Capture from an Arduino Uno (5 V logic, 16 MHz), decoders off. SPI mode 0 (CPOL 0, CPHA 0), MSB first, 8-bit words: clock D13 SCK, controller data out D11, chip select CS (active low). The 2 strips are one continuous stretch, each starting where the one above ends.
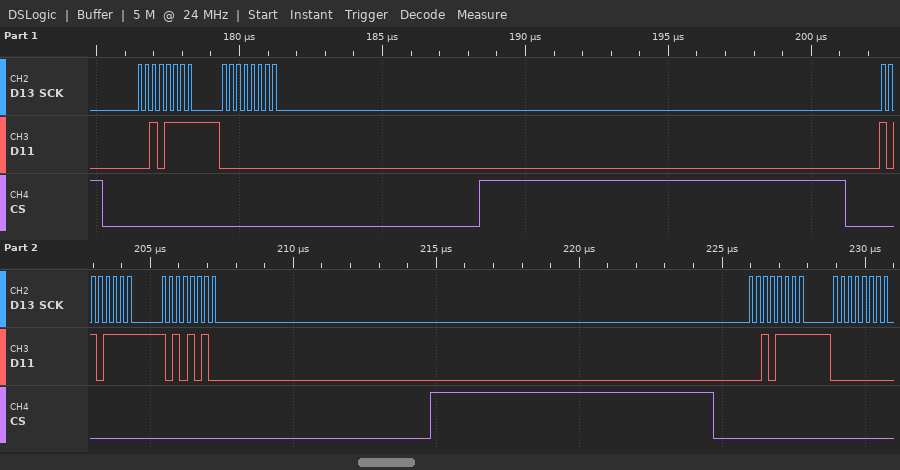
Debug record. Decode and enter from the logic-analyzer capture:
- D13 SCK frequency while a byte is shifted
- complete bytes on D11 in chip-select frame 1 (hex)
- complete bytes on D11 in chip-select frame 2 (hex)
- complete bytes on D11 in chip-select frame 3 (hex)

4 MHz
2F 00
AF AA
2F 00
